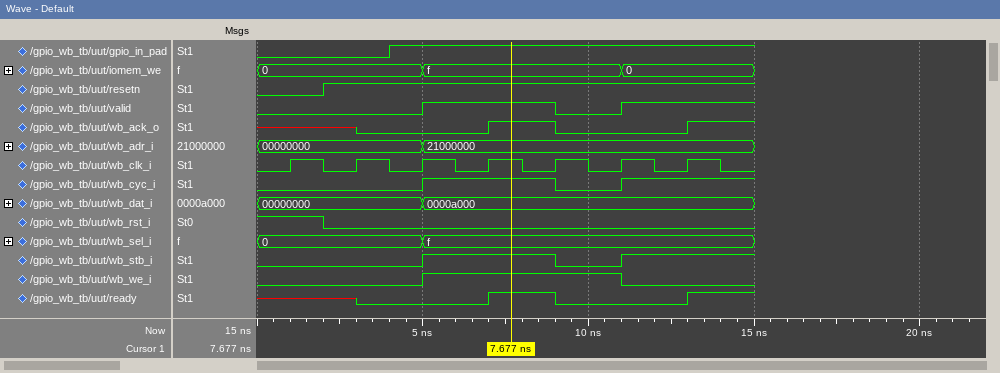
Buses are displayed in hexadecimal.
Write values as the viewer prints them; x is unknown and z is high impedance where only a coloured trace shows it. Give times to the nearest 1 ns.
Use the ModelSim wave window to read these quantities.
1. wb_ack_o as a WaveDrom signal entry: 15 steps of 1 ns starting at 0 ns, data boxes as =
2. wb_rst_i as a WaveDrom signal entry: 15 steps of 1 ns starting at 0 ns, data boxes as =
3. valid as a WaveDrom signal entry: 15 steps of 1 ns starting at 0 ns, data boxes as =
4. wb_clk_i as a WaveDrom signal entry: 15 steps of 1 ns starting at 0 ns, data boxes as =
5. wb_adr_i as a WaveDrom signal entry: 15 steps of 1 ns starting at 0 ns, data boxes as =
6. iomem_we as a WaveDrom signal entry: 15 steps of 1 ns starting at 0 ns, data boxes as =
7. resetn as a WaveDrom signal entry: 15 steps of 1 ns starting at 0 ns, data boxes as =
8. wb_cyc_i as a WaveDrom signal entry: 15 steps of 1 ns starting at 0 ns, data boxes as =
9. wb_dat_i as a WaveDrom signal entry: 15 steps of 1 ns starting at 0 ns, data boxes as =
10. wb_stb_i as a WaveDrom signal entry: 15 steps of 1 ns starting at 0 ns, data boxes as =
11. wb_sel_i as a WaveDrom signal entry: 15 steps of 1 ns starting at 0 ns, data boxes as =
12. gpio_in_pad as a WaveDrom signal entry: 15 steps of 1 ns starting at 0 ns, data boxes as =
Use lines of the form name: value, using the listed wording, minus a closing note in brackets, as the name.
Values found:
wb_ack_o as a WaveDrom signal entry: 15 steps of 1 ns starting at 0 ns, data boxes as =: {name: 'wb_ack_o', wave: 'x..0...1.0...1.'}
wb_rst_i as a WaveDrom signal entry: 15 steps of 1 ns starting at 0 ns, data boxes as =: {name: 'wb_rst_i', wave: '1.0............'}
valid as a WaveDrom signal entry: 15 steps of 1 ns starting at 0 ns, data boxes as =: {name: 'valid', wave: '0....1...0.1...'}
wb_clk_i as a WaveDrom signal entry: 15 steps of 1 ns starting at 0 ns, data boxes as =: {name: 'wb_clk_i', wave: '010101010101010'}
wb_adr_i as a WaveDrom signal entry: 15 steps of 1 ns starting at 0 ns, data boxes as =: {name: 'wb_adr_i', wave: '=....=.........', data: '00000000 21000000'}
iomem_we as a WaveDrom signal entry: 15 steps of 1 ns starting at 0 ns, data boxes as =: {name: 'iomem_we', wave: '=....=.....=...', data: '0 f 0'}
resetn as a WaveDrom signal entry: 15 steps of 1 ns starting at 0 ns, data boxes as =: {name: 'resetn', wave: '0.1............'}
wb_cyc_i as a WaveDrom signal entry: 15 steps of 1 ns starting at 0 ns, data boxes as =: {name: 'wb_cyc_i', wave: '0....1...0.1...'}
wb_dat_i as a WaveDrom signal entry: 15 steps of 1 ns starting at 0 ns, data boxes as =: {name: 'wb_dat_i', wave: '=....=.........', data: '00000000 0000a000'}
wb_stb_i as a WaveDrom signal entry: 15 steps of 1 ns starting at 0 ns, data boxes as =: {name: 'wb_stb_i', wave: '0....1...0.1...'}
wb_sel_i as a WaveDrom signal entry: 15 steps of 1 ns starting at 0 ns, data boxes as =: {name: 'wb_sel_i', wave: '=....=.........', data: '0 f'}
gpio_in_pad as a WaveDrom signal entry: 15 steps of 1 ns starting at 0 ns, data boxes as =: {name: 'gpio_in_pad', wave: '0...1..........'}
